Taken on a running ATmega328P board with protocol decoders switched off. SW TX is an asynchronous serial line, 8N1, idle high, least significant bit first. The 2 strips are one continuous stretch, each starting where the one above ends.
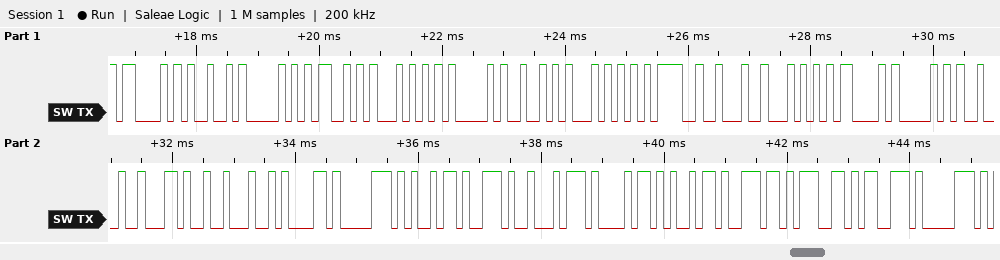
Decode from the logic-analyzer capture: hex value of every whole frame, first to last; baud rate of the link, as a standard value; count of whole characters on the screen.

43 49 50 53 54 41 52 54 3D 22 54 43 50 22 2C 22 61 70 69 2E 74 68 69 6E 67 73 70
9600 baud
27
